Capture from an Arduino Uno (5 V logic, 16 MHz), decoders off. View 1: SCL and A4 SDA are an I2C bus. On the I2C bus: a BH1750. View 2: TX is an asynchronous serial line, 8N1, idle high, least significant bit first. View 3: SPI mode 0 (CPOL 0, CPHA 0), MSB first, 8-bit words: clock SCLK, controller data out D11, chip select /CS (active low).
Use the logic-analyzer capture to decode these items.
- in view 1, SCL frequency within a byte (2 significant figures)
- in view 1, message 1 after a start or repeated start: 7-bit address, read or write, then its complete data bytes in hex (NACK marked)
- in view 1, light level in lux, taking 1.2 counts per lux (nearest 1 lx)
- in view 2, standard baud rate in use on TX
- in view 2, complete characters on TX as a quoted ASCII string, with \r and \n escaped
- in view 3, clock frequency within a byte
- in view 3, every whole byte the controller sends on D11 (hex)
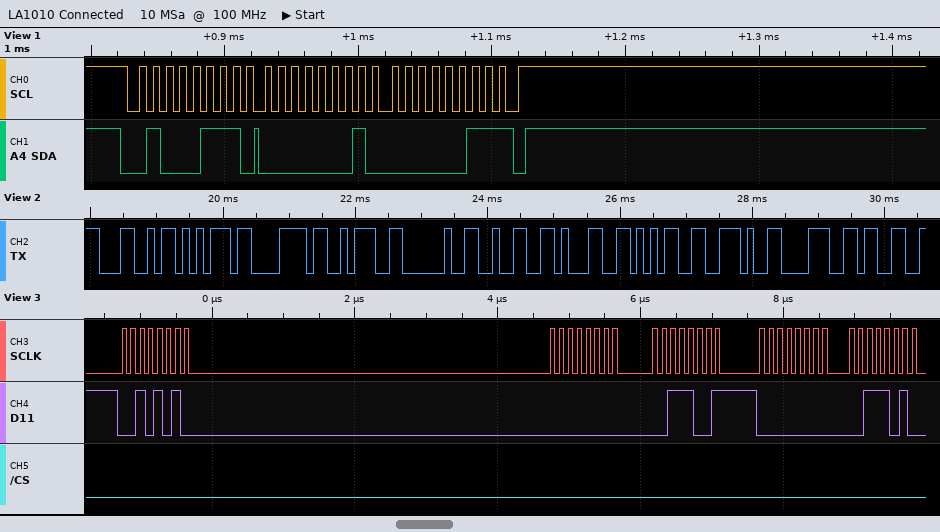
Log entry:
100 kHz
0x23 read: 01 03 NACK
216 lx
9600 baud
"Lux: 215.83"
8 MHz
0x2A 0x00 0x39 0x00 0x3A
